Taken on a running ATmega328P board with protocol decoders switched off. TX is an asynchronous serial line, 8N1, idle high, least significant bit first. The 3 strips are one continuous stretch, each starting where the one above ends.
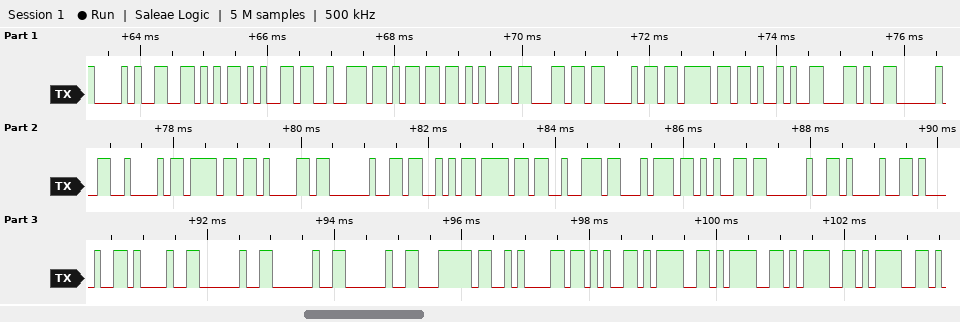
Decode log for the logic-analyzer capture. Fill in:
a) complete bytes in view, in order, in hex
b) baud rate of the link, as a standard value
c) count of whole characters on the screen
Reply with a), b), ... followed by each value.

a) 28 56 65 72 6D 65 6C 68 6F 29 2C 20 42 6F 61 20 53 6F 72 74 65 20 21 21 21 20 20 20 7C 0A 2B 3D 3D 3D 3D
b) 9600 baud
c) 35
